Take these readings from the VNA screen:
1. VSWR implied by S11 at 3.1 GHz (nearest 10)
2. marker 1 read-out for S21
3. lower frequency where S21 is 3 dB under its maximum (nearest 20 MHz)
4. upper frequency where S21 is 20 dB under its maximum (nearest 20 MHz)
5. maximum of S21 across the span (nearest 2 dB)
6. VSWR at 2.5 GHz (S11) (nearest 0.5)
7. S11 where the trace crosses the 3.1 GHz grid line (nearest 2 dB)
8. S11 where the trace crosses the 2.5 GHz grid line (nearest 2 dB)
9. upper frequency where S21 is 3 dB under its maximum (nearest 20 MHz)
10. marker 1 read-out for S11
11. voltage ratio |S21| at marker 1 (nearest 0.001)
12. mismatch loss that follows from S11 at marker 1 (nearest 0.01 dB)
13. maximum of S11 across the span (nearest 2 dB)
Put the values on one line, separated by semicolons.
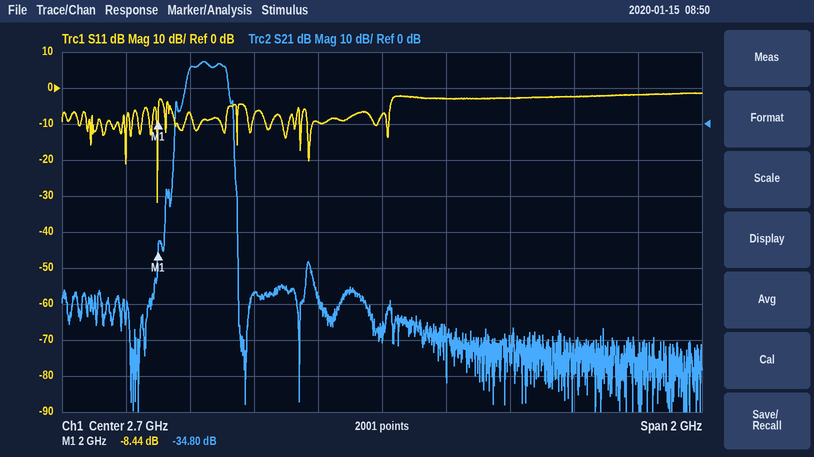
10; -34.80 dB; 2.10 GHz; 2.24 GHz; 18 dB; 2.0; -2 dB; -10 dB; 2.22 GHz; -8.44 dB; 0.018; 0.67 dB; -2 dB
